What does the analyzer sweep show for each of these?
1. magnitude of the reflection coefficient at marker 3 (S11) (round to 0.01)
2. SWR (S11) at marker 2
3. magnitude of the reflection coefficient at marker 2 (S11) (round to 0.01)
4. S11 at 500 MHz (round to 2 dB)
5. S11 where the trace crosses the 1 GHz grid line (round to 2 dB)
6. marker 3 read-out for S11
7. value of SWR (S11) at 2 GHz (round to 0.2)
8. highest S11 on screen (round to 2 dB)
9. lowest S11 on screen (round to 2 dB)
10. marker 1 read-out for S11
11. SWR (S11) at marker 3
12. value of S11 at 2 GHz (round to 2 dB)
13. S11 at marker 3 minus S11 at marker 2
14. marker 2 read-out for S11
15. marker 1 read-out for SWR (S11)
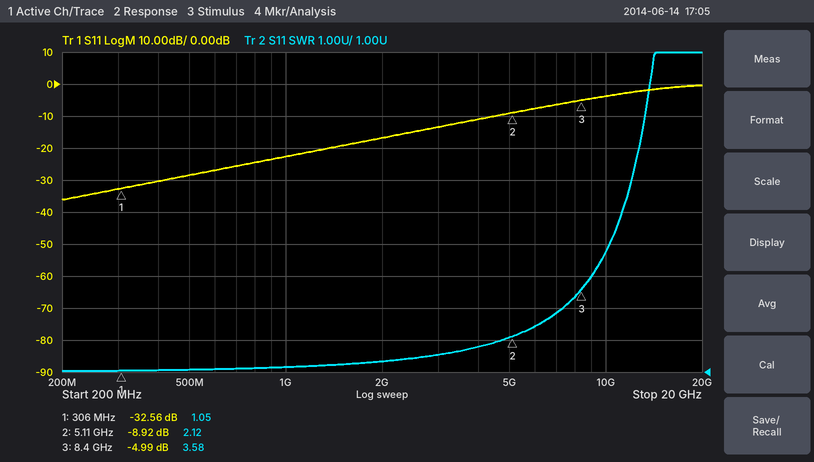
0.56
2.12
0.36
-28 dB
-22 dB
-4.99 dB
1.4
0 dB
-36 dB
-32.56 dB
3.58
-16 dB
3.93 dB
-8.92 dB
1.05
